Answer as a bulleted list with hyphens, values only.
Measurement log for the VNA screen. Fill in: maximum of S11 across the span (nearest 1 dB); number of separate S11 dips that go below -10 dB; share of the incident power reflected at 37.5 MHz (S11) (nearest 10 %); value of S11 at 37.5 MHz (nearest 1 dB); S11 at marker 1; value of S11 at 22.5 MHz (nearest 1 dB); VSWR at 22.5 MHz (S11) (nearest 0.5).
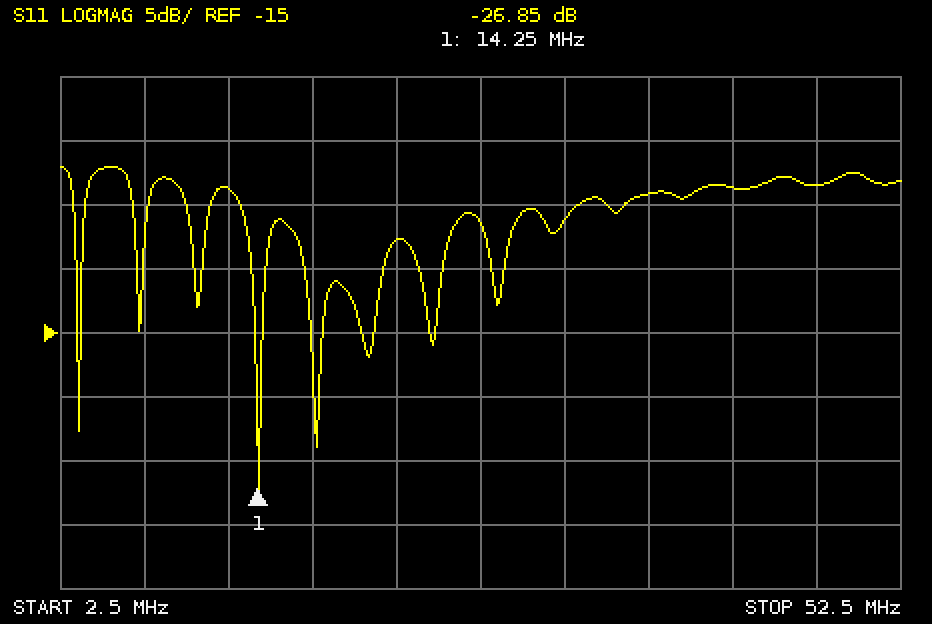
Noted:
- -2 dB
- 8
- 40 %
- -4 dB
- -26.85 dB
- -8 dB
- 2.5
